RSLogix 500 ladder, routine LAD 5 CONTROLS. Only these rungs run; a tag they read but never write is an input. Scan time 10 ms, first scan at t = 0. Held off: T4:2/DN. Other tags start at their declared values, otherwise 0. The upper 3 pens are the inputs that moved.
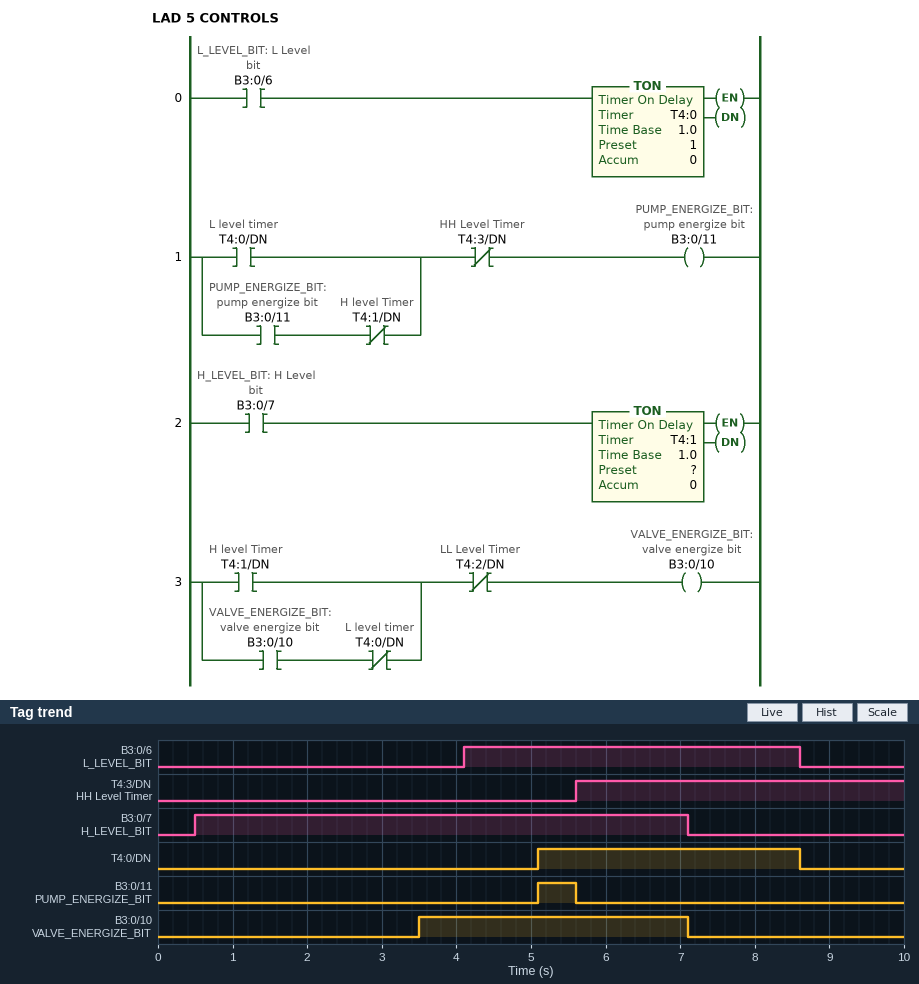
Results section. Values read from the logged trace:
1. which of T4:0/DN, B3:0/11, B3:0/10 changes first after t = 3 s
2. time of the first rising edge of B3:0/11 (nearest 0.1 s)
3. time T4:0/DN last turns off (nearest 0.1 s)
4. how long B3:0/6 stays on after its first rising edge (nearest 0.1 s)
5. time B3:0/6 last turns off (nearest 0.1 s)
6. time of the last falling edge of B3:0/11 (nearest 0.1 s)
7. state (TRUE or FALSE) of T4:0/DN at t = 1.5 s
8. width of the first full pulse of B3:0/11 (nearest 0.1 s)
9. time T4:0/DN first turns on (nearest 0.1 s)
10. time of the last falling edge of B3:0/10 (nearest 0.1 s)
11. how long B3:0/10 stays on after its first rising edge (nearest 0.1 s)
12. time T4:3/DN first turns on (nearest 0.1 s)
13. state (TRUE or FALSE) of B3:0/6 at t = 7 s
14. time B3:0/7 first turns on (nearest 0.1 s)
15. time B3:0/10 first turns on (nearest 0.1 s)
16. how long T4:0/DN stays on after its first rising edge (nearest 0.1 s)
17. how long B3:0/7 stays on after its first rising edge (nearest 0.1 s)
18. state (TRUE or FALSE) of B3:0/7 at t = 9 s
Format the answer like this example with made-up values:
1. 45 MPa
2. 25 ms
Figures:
1. B3:0/10
2. 5.1 s
3. 8.6 s
4. 4.5 s
5. 8.6 s
6. 5.6 s
7. FALSE
8. 0.5 s
9. 5.1 s
10. 7.1 s
11. 3.6 s
12. 5.6 s
13. TRUE
14. 0.5 s
15. 3.5 s
16. 3.5 s
17. 6.6 s
18. FALSE
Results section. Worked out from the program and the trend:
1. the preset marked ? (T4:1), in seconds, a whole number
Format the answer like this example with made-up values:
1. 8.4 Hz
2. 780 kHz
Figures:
1. 3 s
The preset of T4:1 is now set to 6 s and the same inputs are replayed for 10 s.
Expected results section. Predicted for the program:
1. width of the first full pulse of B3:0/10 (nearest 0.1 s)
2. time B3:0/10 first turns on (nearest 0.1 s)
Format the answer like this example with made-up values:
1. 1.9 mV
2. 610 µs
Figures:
1. 0.6 s
2. 6.5 s
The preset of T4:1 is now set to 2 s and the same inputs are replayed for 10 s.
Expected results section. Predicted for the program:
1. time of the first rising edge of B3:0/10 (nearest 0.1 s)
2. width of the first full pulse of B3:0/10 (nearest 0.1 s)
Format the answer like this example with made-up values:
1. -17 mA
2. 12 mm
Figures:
1. 2.5 s
2. 4.6 s
